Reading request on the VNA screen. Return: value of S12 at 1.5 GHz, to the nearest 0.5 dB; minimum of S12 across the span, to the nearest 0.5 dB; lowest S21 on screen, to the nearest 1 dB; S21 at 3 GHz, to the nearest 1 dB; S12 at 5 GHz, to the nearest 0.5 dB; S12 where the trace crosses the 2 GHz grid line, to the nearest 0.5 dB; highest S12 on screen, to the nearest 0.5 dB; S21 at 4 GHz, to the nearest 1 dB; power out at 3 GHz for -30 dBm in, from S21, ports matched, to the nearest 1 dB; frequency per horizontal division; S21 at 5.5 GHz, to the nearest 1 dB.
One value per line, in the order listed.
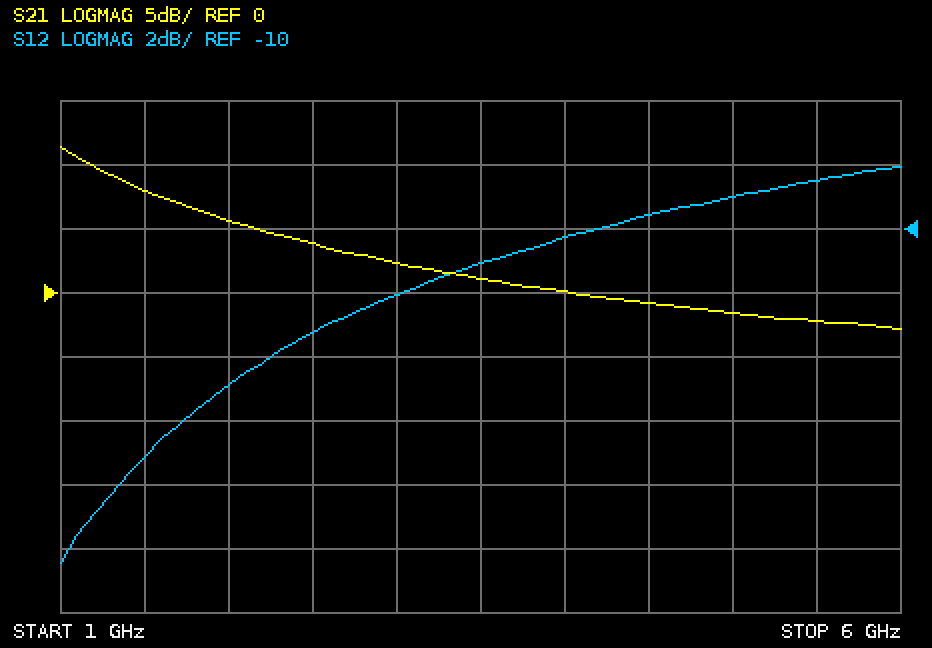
-17.0 dB
-20.5 dB
-3 dB
2 dB
-9.0 dB
-15.0 dB
-8.0 dB
0 dB
-28 dBm
500 MHz
-2 dB
